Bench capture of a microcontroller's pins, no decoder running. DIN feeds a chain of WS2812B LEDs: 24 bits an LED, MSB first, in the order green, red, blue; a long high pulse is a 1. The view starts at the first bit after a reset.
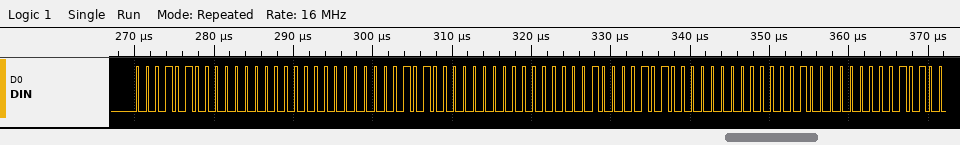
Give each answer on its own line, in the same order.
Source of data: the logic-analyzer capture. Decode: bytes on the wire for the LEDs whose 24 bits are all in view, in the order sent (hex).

14 00 00 14 00 02 14 00 10
